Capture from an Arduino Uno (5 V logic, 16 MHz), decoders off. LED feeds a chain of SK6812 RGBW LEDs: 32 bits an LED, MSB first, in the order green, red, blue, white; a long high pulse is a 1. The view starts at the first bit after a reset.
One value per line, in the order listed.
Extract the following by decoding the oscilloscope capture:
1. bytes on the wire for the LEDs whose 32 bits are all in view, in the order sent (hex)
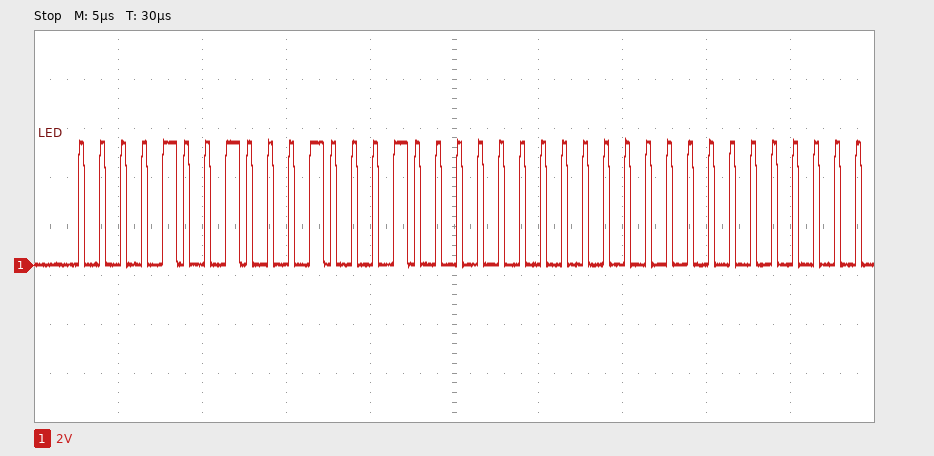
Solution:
09 11 00 00
